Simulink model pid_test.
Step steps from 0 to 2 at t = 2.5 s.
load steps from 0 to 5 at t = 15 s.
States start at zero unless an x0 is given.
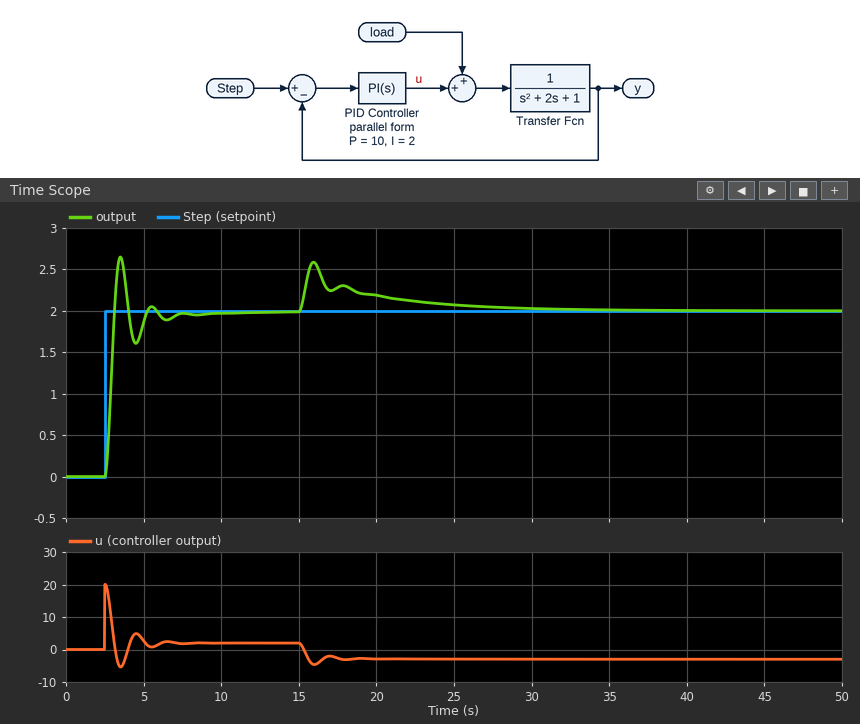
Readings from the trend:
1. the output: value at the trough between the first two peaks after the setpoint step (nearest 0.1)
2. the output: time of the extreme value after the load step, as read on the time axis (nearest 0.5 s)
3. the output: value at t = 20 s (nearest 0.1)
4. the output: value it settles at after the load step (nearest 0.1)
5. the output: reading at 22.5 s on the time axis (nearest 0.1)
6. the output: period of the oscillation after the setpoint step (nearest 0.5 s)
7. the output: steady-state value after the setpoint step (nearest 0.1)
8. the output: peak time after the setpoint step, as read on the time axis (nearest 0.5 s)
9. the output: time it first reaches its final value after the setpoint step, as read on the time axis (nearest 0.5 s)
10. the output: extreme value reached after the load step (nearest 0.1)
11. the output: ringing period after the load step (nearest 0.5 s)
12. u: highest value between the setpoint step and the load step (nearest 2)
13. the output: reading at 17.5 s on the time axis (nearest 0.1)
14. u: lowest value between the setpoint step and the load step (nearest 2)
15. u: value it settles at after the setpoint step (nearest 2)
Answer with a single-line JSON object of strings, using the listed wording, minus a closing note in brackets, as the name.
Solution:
{"the output: value at the trough between the first two peaks after the setpoint step": "1.6", "the output: time of the extreme value after the load step, as read on the time axis": "16.0 s", "the output: value at t = 20 s": "2.2", "the output: value it settles at after the load step": "2.0", "the output: reading at 22.5 s on the time axis": "2.1", "the output: period of the oscillation after the setpoint step": "2.0 s", "the output: steady-state value after the setpoint step": "2.0", "the output: peak time after the setpoint step, as read on the time axis": "3.5 s", "the output: time it first reaches its final value after the setpoint step, as read on the time axis": "3.0 s", "the output: extreme value reached after the load step": "2.6", "the output: ringing period after the load step": "2.0 s", "u: highest value between the setpoint step and the load step": "20", "the output: reading at 17.5 s on the time axis": "2.3", "u: lowest value between the setpoint step and the load step": "-6", "u: value it settles at after the setpoint step": "2"}
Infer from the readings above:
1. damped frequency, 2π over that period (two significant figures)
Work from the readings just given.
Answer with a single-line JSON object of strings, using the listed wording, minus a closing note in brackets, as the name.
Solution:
{"damped frequency, 2π over that period": "3.1 rad/s"}
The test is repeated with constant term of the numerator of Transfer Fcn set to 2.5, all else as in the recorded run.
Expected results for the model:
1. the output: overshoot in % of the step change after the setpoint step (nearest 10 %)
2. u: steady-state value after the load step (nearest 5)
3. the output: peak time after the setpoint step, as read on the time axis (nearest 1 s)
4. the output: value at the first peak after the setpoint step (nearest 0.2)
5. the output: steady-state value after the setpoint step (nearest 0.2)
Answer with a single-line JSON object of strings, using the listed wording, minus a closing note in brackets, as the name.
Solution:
{"the output: overshoot in % of the step change after the setpoint step": "50 %", "u: steady-state value after the load step": "-5", "the output: peak time after the setpoint step, as read on the time axis": "3 s", "the output: value at the first peak after the setpoint step": "3.0", "the output: steady-state value after the setpoint step": "2.0"}
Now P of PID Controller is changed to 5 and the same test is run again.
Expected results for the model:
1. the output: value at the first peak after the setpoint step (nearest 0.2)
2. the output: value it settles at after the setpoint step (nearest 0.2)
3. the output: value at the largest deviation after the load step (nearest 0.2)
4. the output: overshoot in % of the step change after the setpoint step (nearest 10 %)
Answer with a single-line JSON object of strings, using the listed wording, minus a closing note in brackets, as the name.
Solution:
{"the output: value at the first peak after the setpoint step": "2.4", "the output: value it settles at after the setpoint step": "2.0", "the output: value at the largest deviation after the load step": "3.0", "the output: overshoot in % of the step change after the setpoint step": "20 %"}
